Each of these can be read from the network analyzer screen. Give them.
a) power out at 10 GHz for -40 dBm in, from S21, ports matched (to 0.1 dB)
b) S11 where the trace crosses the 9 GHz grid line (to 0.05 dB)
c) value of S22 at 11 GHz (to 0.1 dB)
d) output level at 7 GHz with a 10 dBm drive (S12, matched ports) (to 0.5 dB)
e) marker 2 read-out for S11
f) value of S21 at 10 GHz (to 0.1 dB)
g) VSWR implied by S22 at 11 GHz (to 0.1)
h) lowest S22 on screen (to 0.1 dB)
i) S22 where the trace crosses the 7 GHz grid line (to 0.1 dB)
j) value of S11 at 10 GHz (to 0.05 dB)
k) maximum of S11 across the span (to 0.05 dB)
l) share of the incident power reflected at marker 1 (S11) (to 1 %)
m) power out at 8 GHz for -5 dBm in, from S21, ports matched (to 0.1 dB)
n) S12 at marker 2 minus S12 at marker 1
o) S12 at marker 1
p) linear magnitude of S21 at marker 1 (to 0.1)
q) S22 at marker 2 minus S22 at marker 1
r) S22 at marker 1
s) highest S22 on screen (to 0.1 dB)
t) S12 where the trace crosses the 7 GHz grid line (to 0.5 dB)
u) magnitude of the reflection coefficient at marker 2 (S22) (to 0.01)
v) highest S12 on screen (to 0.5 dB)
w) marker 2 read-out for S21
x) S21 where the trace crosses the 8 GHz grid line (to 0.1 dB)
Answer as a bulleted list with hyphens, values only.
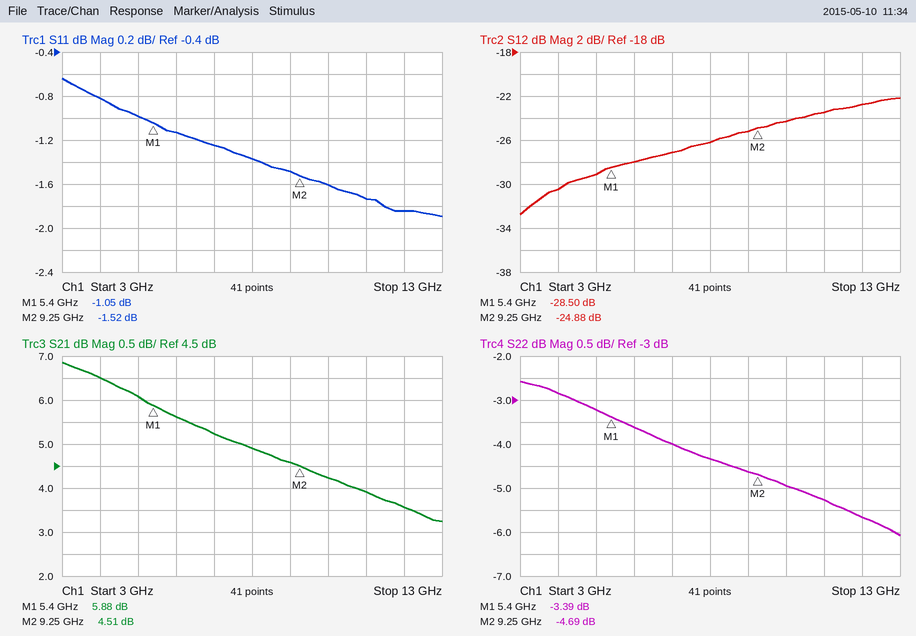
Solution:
- -35.8 dBm
- -1.50 dB
- -5.3 dB
- -17.0 dBm
- -1.52 dB
- 4.2 dB
- 3.4
- -6.1 dB
- -4.0 dB
- -1.60 dB
- -0.65 dB
- 79 %
- -0.1 dBm
- 3.62 dB
- -28.50 dB
- 2.0
- -1.30 dB
- -3.39 dB
- -2.6 dB
- -27.0 dB
- 0.58
- -22.0 dB
- 4.51 dB
- 4.9 dB
